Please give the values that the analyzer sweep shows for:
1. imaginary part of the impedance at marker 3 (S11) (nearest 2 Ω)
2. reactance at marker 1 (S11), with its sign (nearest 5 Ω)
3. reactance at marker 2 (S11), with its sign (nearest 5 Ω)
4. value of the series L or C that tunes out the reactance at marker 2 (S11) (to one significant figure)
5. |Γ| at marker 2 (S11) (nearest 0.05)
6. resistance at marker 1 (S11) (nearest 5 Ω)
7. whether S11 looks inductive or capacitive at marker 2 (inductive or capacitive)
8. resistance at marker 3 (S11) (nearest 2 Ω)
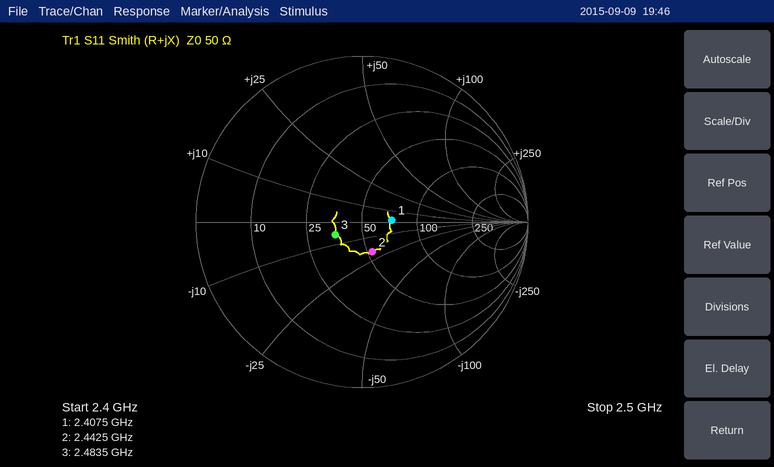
-6 Ω
0 Ω
-20 Ω
1 nH
0.20
70 Ω
capacitive
36 Ω
